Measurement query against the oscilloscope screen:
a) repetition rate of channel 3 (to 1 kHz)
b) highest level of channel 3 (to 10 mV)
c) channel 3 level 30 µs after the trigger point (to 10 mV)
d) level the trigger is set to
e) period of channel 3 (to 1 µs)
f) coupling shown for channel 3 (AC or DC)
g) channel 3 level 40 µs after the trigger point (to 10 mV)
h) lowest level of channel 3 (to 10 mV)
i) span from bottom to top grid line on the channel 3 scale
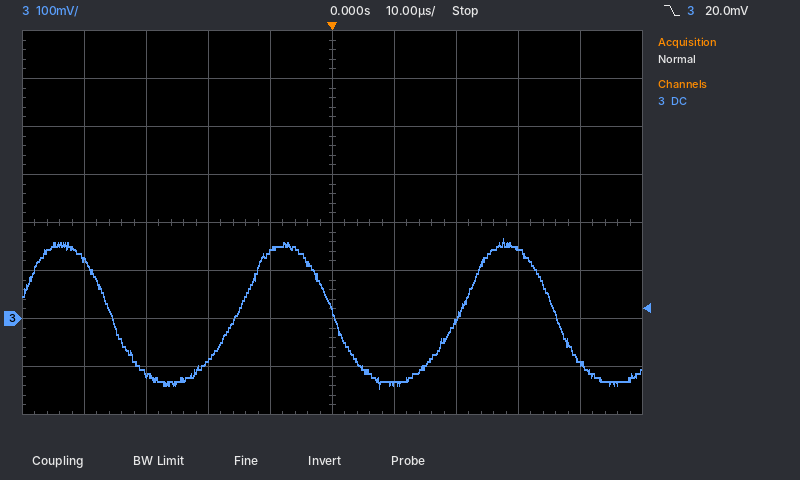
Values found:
28 kHz
170 mV
150 mV
20.0 mV
36 µs
DC
-90 mV
-150 mV
800 mV
